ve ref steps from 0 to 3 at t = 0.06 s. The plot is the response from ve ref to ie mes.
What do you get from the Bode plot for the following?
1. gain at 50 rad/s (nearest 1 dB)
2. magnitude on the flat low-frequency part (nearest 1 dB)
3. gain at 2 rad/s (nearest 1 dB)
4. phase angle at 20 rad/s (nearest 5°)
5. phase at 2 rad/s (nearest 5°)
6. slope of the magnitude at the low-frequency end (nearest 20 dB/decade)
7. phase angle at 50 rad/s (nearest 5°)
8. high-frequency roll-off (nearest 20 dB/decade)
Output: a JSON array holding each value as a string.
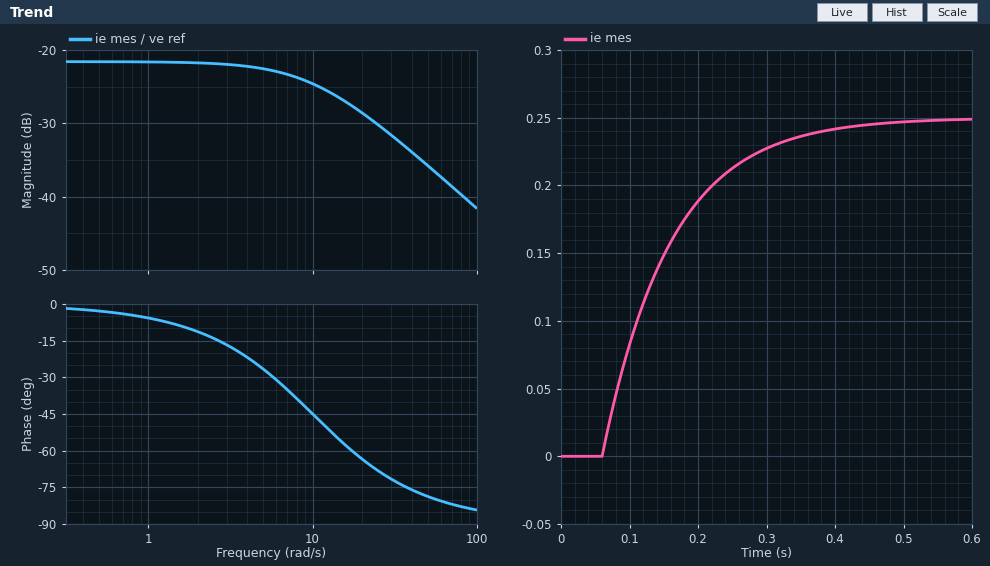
["-36 dB", "-22 dB", "-22 dB", "-65°", "-10°", "0 dB/decade", "-80°", "-20 dB/decade"]
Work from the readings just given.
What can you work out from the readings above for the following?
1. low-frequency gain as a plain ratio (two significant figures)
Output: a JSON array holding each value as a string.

["0.079"]
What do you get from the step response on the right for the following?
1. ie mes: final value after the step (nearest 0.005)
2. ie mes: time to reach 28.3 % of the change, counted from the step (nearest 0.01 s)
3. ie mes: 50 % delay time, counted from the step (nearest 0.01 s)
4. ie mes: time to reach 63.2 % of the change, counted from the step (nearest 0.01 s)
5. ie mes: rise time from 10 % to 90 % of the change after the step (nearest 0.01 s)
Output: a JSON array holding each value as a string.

["0.250", "0.03 s", "0.07 s", "0.10 s", "0.22 s"]
